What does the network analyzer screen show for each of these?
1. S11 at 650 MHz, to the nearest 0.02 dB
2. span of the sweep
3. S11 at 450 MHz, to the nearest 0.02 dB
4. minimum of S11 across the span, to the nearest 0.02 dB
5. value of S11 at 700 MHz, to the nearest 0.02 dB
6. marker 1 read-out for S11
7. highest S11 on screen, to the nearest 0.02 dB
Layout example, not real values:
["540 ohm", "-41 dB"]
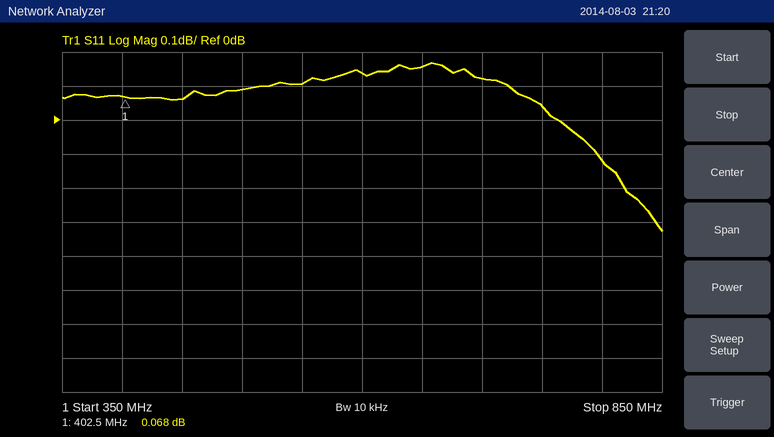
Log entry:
["0.16 dB", "500 MHz", "0.06 dB", "-0.32 dB", "0.12 dB", "0.068 dB", "0.16 dB"]
